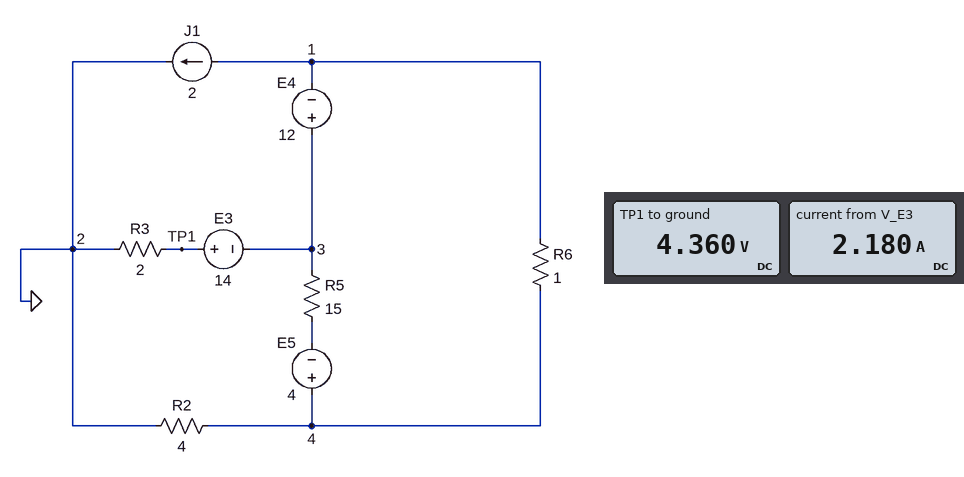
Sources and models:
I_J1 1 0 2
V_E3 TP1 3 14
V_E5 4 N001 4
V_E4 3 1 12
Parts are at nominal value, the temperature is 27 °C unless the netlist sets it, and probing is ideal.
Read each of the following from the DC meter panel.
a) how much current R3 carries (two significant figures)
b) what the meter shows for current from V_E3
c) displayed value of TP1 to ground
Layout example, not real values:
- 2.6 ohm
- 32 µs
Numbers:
- 2.2 A
- 2.180 A
- 4.360 V
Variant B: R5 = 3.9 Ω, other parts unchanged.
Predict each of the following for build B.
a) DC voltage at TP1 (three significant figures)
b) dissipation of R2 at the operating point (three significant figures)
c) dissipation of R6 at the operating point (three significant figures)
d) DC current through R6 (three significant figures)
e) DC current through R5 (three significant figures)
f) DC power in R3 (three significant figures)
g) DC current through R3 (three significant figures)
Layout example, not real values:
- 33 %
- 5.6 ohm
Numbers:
- 3.87 V
- 61.9 W
- 40.9 W
- 6.40 A
- 2.46 A
- 7.48 W
- 1.93 A
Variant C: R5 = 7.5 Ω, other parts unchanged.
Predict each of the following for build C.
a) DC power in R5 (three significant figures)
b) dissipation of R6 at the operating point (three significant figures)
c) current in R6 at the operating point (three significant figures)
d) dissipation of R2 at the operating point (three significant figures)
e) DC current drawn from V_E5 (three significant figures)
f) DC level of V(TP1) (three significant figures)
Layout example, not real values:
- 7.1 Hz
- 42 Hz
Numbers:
- 14.7 W
- 30.1 W
- 5.49 A
- 66.8 W
- 1.40 A
- 4.17 V
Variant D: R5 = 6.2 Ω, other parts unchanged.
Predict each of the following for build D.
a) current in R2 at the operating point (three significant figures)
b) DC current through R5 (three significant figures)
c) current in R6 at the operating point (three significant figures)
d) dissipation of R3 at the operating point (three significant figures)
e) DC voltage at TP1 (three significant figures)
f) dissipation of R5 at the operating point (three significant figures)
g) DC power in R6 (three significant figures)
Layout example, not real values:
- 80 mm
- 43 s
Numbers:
- 4.05 A
- 1.66 A
- 5.71 A
- 8.39 W
- 4.10 V
- 17.1 W
- 32.6 W
